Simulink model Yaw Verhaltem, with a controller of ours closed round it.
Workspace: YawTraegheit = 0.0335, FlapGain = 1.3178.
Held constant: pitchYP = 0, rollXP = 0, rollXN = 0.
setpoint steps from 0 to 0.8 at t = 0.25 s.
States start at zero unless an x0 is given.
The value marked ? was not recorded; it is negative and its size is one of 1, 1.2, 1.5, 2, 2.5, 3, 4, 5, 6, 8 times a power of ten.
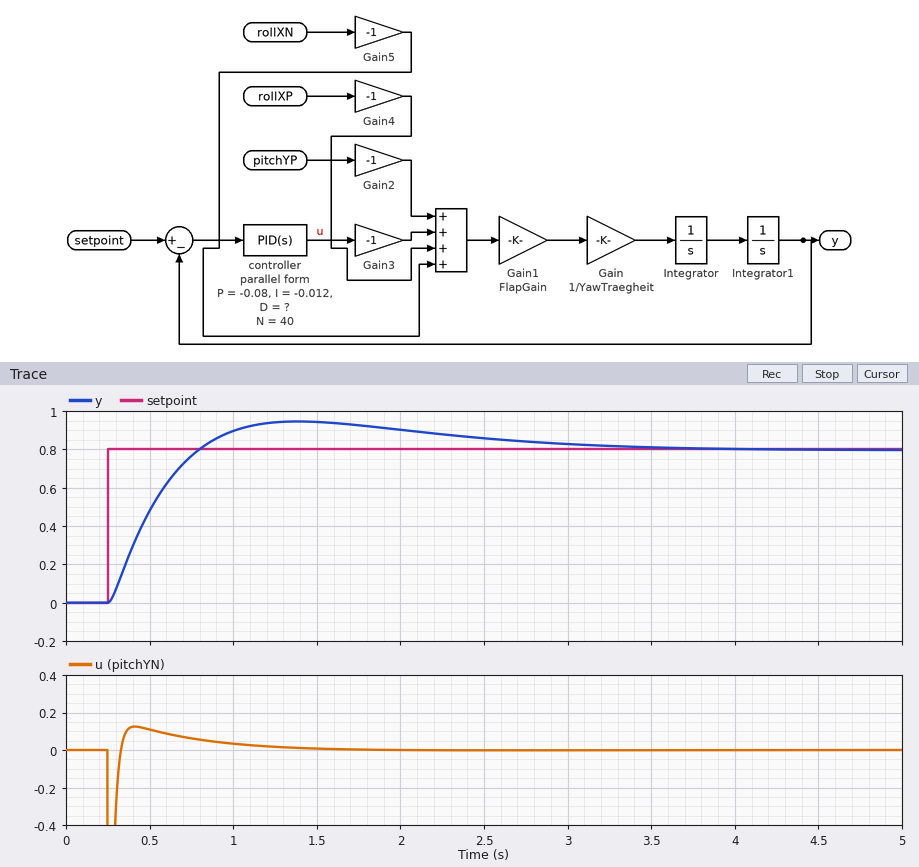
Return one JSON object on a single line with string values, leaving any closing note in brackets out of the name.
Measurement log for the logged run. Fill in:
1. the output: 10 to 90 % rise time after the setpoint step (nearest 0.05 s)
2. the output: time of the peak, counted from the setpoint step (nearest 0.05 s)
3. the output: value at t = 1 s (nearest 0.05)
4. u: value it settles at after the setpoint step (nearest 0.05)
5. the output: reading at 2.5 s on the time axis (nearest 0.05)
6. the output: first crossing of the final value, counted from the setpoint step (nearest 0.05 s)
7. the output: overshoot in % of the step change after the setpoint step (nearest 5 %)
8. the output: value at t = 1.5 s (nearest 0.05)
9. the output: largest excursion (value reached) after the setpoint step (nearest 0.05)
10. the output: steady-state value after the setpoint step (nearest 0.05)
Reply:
{"the output: 10 to 90 % rise time after the setpoint step": "0.40 s", "the output: time of the peak, counted from the setpoint step": "1.15 s", "the output: value at t = 1 s": "0.90", "u: value it settles at after the setpoint step": "0.00", "the output: reading at 2.5 s on the time axis": "0.85", "the output: first crossing of the final value, counted from the setpoint step": "0.55 s", "the output: overshoot in % of the step change after the setpoint step": "20 %", "the output: value at t = 1.5 s": "0.95", "the output: largest excursion (value reached) after the setpoint step": "0.95", "the output: steady-state value after the setpoint step": "0.80"}
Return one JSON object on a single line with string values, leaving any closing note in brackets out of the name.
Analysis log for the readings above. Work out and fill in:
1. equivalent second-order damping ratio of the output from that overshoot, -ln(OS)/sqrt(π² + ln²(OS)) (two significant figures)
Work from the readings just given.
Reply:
{"equivalent second-order damping ratio of the output from that overshoot, -ln(OS)/sqrt(π² + ln²(OS))": "0.46"}
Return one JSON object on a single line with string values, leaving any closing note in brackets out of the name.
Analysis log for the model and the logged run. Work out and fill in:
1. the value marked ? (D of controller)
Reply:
{"the value marked ?": "-0.08"}
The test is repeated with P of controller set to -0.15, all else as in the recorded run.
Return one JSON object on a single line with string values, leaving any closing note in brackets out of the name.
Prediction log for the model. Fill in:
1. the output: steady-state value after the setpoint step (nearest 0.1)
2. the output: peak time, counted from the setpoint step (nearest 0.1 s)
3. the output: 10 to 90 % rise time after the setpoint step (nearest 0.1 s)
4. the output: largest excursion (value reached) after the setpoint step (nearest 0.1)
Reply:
{"the output: steady-state value after the setpoint step": "0.8", "the output: peak time, counted from the setpoint step": "0.9 s", "the output: 10 to 90 % rise time after the setpoint step": "0.3 s", "the output: largest excursion (value reached) after the setpoint step": "1.0"}
